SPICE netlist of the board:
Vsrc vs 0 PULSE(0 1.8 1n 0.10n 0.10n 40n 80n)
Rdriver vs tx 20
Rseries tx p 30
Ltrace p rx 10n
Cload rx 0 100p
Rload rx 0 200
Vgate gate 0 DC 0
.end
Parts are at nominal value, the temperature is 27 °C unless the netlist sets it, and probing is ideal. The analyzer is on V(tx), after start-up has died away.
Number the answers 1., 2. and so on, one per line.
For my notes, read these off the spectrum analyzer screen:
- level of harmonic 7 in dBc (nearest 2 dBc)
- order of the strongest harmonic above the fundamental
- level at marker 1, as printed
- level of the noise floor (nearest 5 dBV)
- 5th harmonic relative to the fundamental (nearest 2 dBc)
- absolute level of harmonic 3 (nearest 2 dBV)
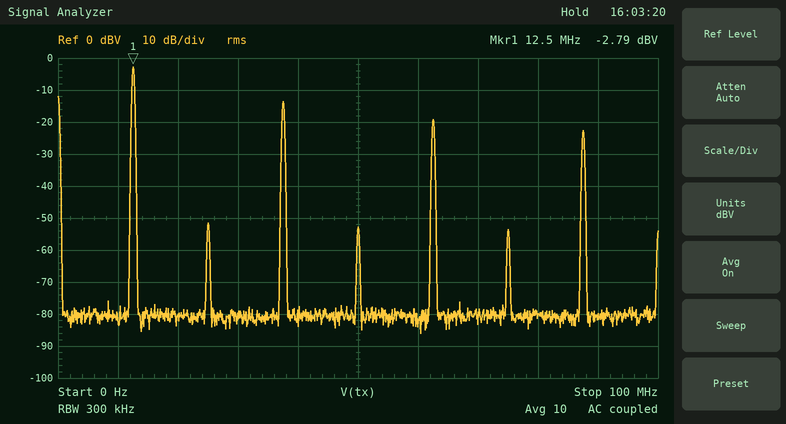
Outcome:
1. -20 dBc
2. 3
3. -2.79 dBV
4. -80 dBV
5. -16 dBc
6. -14 dBV
